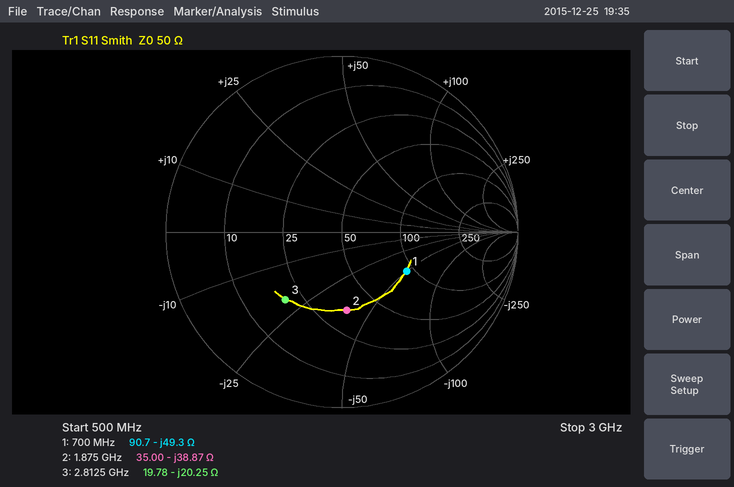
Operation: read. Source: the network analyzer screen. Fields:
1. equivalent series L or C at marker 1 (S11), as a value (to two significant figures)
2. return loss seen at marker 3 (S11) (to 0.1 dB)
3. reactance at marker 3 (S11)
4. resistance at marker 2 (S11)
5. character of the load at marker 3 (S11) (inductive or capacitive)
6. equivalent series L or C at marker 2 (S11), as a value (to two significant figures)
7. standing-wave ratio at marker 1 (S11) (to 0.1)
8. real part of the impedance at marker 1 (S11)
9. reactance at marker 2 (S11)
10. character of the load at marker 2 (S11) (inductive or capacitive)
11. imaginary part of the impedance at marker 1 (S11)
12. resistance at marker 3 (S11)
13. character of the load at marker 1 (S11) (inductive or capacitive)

4.6 pF
6.0 dB
-20.25 Ω
35.00 Ω
capacitive
2.2 pF
2.5
90.7 Ω
-38.87 Ω
capacitive
-49.3 Ω
19.78 Ω
capacitive
